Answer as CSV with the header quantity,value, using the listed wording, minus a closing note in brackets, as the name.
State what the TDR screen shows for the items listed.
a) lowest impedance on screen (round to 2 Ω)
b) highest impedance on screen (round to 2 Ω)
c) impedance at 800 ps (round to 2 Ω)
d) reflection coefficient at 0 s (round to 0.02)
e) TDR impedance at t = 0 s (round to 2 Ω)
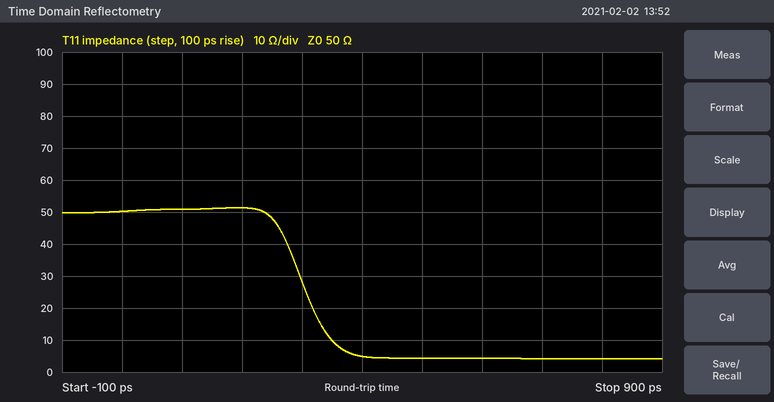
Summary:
quantity,value
lowest impedance on screen,4 Ω
highest impedance on screen,52 Ω
impedance at 800 ps,4 Ω
reflection coefficient at 0 s,0.00
TDR impedance at t = 0 s,50 Ω
